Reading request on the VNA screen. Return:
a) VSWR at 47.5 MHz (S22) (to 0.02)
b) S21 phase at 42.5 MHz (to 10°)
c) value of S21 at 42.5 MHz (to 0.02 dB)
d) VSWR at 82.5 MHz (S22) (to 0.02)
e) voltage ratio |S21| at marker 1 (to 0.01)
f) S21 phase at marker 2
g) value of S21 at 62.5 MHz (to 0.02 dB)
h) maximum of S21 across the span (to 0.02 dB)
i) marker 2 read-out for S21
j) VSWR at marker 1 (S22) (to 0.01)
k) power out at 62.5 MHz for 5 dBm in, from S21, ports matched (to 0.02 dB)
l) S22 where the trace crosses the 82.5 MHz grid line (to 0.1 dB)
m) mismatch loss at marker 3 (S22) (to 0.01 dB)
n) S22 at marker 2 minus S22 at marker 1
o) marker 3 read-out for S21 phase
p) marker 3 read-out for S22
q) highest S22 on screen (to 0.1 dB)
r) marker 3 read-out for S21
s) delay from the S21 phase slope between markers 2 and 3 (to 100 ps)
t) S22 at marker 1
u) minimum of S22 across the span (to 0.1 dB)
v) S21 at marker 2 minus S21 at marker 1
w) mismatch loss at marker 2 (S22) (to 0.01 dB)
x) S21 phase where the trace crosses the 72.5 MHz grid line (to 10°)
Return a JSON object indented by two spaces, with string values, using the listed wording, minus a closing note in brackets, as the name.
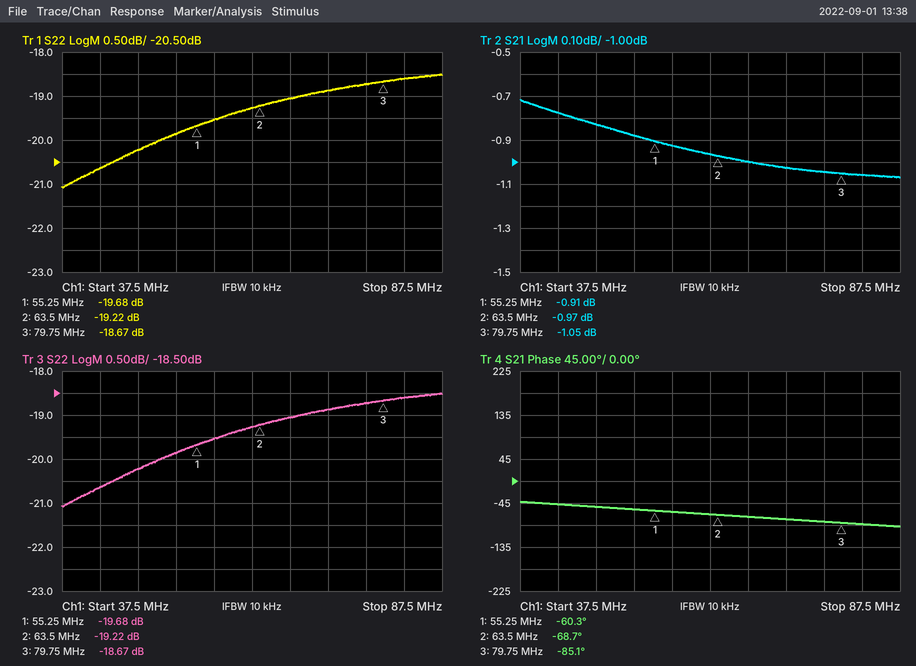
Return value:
{
  "VSWR at 47.5 MHz (S22)": "1.22",
  "S21 phase at 42.5 MHz": "-50°",
  "value of S21 at 42.5 MHz": "-0.78 dB",
  "VSWR at 82.5 MHz (S22)": "1.26",
  "voltage ratio |S21| at marker 1": "0.90",
  "S21 phase at marker 2": "-68.7°",
  "value of S21 at 62.5 MHz": "-0.96 dB",
  "maximum of S21 across the span": "-0.72 dB",
  "marker 2 read-out for S21": "-0.97 dB",
  "VSWR at marker 1 (S22)": "1.23",
  "power out at 62.5 MHz for 5 dBm in, from S21, ports matched": "4.04 dBm",
  "S22 where the trace crosses the 82.5 MHz grid line": "-18.6 dB",
  "mismatch loss at marker 3 (S22)": "0.06 dB",
  "S22 at marker 2 minus S22 at marker 1": "0.46 dB",
  "marker 3 read-out for S21 phase": "-85.1°",
  "marker 3 read-out for S22": "-18.67 dB",
  "highest S22 on screen": "-18.5 dB",
  "marker 3 read-out for S21": "-1.05 dB",
  "delay from the S21 phase slope between markers 2 and 3": "2.8 ns",
  "S22 at marker 1": "-19.68 dB",
  "minimum of S22 across the span": "-21.1 dB",
  "S21 at marker 2 minus S21 at marker 1": "-0.06 dB",
  "mismatch loss at marker 2 (S22)": "0.05 dB",
  "S21 phase where the trace crosses the 72.5 MHz grid line": "-80°"
}
